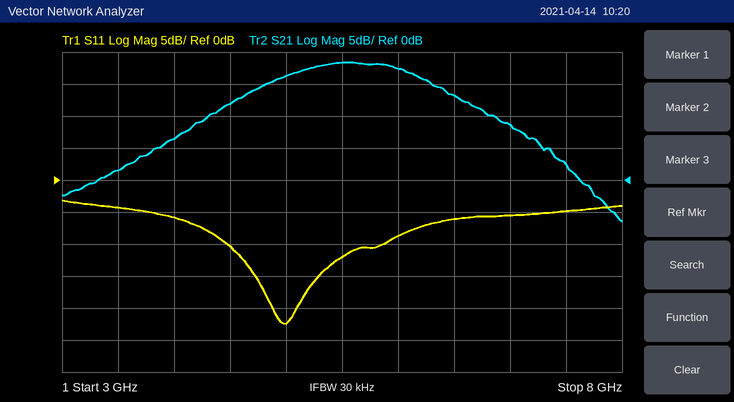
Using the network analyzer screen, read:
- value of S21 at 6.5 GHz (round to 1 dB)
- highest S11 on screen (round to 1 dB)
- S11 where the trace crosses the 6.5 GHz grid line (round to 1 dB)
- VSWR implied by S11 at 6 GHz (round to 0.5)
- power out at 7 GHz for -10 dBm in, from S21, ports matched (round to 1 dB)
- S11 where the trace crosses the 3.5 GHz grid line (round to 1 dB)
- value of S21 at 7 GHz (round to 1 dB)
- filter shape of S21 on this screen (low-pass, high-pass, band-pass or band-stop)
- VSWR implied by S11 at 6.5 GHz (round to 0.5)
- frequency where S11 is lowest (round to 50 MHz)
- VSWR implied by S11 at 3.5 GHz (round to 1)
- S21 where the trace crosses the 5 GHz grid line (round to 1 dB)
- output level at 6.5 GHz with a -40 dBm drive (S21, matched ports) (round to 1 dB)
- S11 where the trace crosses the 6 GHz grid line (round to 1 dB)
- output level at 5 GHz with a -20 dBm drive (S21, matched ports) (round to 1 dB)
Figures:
13 dB
-3 dB
-6 dB
2.0
-1 dBm
-4 dB
9 dB
band-pass
3.0
5.00 GHz
4
16 dB
-27 dBm
-9 dB
-4 dBm
